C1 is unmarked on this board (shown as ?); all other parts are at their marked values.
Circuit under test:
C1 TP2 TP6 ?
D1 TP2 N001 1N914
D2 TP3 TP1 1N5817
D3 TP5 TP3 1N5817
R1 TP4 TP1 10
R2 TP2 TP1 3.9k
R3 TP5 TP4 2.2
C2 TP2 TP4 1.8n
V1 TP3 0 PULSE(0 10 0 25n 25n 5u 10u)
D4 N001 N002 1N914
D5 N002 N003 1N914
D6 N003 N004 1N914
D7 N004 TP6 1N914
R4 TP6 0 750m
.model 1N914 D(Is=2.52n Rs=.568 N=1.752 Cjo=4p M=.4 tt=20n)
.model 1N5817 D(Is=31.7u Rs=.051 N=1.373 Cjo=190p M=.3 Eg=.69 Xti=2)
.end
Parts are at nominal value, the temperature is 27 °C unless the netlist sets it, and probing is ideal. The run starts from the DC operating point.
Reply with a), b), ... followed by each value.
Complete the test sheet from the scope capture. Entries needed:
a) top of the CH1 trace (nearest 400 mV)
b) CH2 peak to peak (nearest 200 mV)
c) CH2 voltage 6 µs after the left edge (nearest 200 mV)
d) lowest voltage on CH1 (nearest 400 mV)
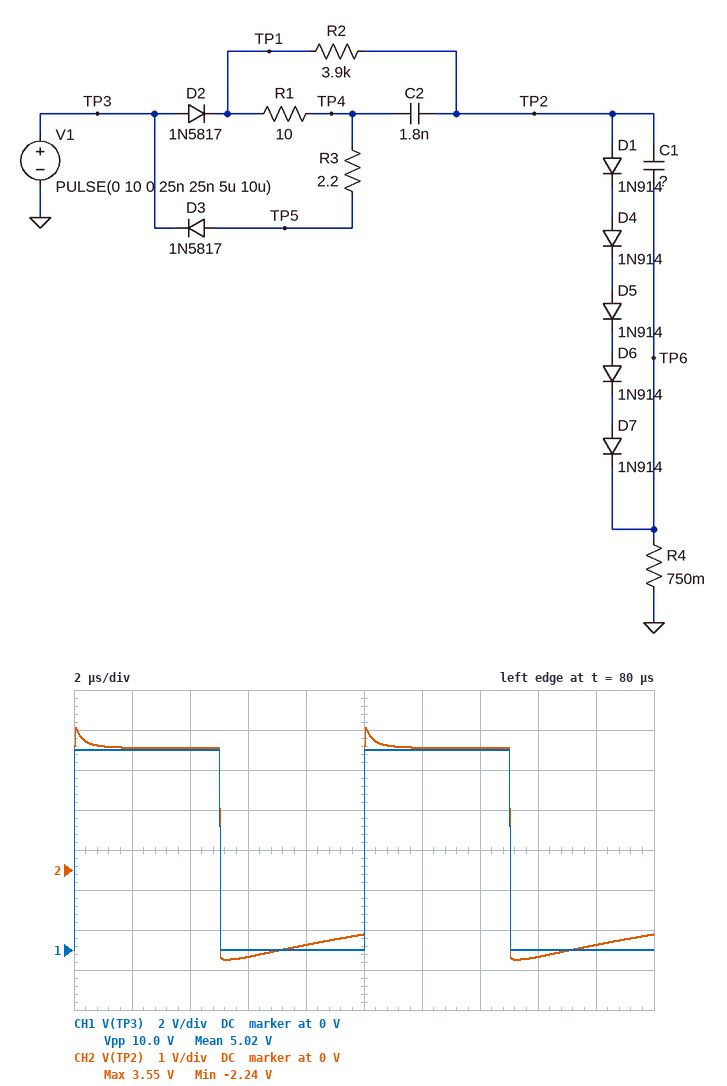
a) 10.0 V
b) 5.8 V
c) -2.2 V
d) 0 V
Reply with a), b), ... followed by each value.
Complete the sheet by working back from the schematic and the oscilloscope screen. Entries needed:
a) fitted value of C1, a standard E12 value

a) 1.5 nF
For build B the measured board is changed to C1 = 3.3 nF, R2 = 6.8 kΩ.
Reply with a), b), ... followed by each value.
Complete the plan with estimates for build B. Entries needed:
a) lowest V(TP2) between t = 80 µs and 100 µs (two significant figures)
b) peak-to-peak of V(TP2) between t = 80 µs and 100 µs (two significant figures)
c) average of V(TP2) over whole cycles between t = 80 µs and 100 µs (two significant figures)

a) -530 mV
b) 3.5 V
c) 1.2 V
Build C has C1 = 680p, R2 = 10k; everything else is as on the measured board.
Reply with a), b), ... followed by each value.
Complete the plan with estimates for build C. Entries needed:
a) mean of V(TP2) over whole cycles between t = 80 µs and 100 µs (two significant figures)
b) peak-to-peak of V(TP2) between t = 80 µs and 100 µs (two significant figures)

a) -500 mV
b) 7.7 V
